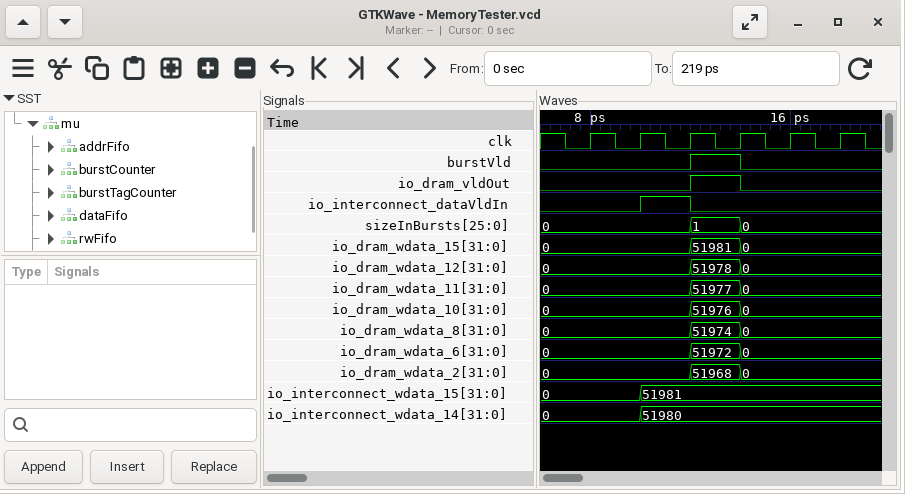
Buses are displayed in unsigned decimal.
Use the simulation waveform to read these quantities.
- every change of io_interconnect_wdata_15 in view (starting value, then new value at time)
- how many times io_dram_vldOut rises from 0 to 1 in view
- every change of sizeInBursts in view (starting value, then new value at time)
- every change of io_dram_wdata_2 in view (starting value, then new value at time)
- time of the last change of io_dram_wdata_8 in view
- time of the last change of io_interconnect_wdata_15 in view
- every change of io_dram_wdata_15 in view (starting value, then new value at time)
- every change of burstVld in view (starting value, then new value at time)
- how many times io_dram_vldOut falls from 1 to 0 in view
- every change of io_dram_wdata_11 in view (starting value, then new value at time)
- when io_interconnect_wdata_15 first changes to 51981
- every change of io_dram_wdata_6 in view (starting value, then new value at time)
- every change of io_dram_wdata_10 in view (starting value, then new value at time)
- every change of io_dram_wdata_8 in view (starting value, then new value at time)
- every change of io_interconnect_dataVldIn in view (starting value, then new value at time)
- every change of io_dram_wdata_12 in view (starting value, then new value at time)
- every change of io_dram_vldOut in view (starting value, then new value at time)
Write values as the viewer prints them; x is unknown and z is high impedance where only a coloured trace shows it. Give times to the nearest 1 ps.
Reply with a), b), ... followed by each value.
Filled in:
a) 0, 51981 at 10 ps
b) 1
c) 0, 1 at 12 ps, 0 at 14 ps
d) 0, 51968 at 12 ps, 0 at 14 ps
e) 14 ps
f) 10 ps
g) 0, 51981 at 12 ps, 0 at 14 ps
h) 0, 1 at 12 ps, 0 at 14 ps
i) 1
j) 0, 51977 at 12 ps, 0 at 14 ps
k) 10 ps
l) 0, 51972 at 12 ps, 0 at 14 ps
m) 0, 51976 at 12 ps, 0 at 14 ps
n) 0, 51974 at 12 ps, 0 at 14 ps
o) 0, 1 at 10 ps, 0 at 12 ps
p) 0, 51978 at 12 ps, 0 at 14 ps
q) 0, 1 at 12 ps, 0 at 14 ps
